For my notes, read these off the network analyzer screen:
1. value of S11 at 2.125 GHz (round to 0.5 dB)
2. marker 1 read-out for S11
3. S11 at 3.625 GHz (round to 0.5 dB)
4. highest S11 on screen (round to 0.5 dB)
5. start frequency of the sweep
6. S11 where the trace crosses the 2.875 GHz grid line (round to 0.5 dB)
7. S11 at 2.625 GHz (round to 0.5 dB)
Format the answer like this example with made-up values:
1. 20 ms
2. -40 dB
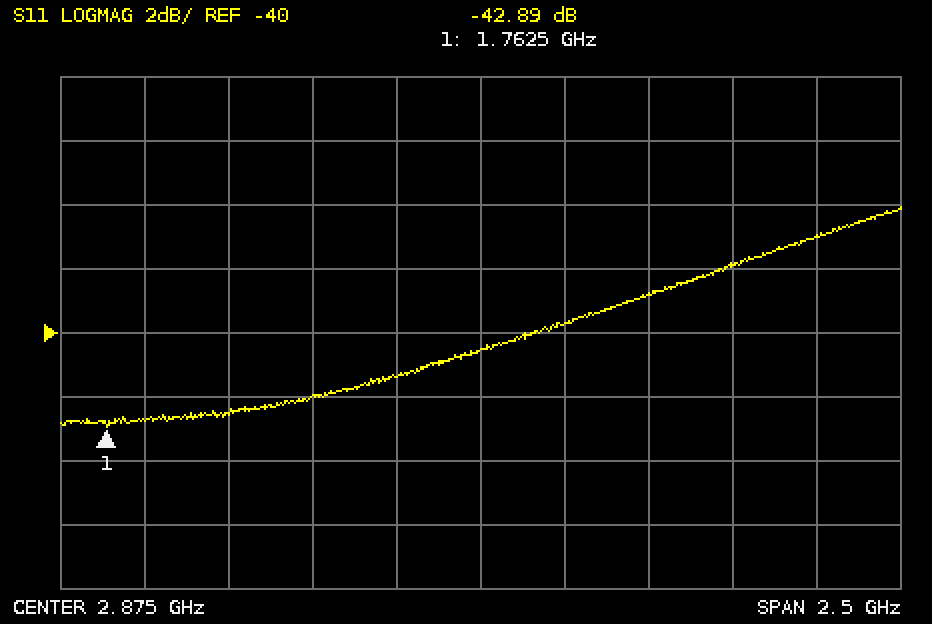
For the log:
1. -42.5 dB
2. -42.89 dB
3. -38.0 dB
4. -36.0 dB
5. 1.625 GHz
6. -40.5 dB
7. -41.5 dB
